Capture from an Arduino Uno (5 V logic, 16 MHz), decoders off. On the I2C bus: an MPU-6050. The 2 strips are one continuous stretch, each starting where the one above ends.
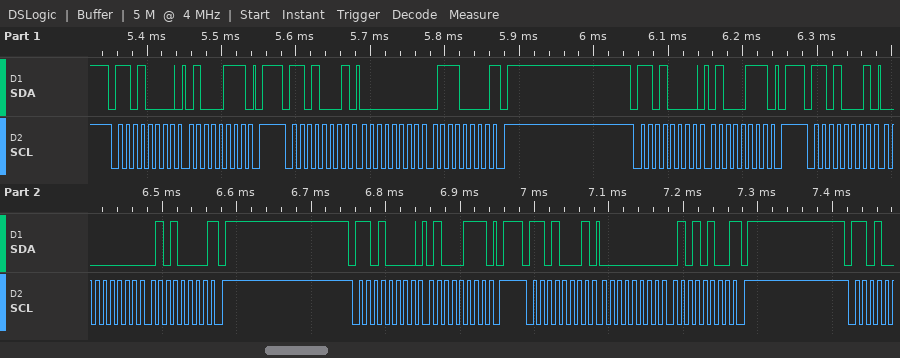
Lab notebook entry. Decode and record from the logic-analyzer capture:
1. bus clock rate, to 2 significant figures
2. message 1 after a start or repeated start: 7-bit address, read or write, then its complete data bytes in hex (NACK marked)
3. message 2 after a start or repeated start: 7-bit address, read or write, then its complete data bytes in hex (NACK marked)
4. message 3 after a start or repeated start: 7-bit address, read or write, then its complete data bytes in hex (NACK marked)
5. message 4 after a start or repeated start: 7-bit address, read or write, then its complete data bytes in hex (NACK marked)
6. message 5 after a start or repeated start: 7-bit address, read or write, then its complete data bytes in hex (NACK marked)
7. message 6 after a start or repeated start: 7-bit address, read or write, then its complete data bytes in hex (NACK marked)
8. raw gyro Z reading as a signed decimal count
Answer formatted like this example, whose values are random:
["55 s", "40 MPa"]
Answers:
["100 kHz", "0x68 write: 47", "0x68 read: 00 70 NACK", "0x68 write: 47", "0x68 read: 00 50 NACK", "0x68 write: 47", "0x68 read: 00 54 NACK", "112"]
